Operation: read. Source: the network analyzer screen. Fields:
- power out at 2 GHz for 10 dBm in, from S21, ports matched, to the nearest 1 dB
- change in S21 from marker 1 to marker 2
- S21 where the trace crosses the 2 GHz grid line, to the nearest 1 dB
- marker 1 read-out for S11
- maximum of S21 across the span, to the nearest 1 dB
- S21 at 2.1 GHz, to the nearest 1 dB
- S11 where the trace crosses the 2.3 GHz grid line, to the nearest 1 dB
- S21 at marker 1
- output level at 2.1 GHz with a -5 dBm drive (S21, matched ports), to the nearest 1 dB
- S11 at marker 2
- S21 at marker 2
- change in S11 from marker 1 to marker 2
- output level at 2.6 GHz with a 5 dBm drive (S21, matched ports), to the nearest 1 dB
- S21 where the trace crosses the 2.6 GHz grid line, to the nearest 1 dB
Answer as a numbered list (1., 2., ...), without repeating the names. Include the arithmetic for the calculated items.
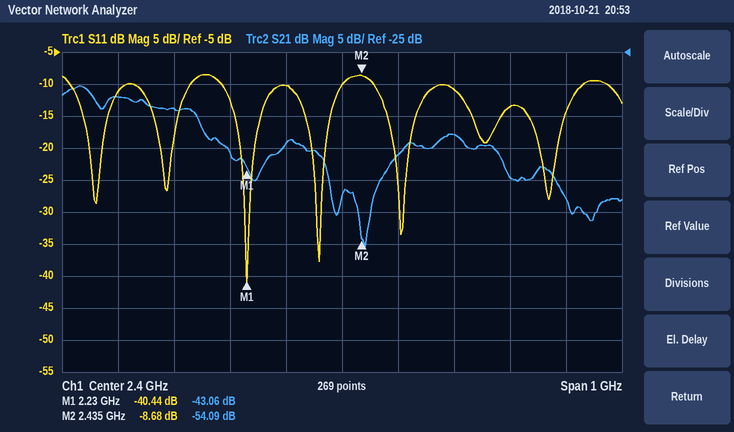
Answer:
1. 10 dBm + (-32 dB) = -22 dBm
2. -54.09 − (-43.06) = -11.03 dB
3. -32 dB
4. -40.44 dB
5. -30 dB
6. -34 dB
7. -10 dB
8. -43.06 dB
9. -5 dBm + (-34 dB) = -39 dBm
10. -8.68 dB
11. -54.09 dB
12. -8.68 − (-40.44) = 31.76 dB
13. 5 dBm + (-38 dB) = -33 dBm
14. -38 dB
